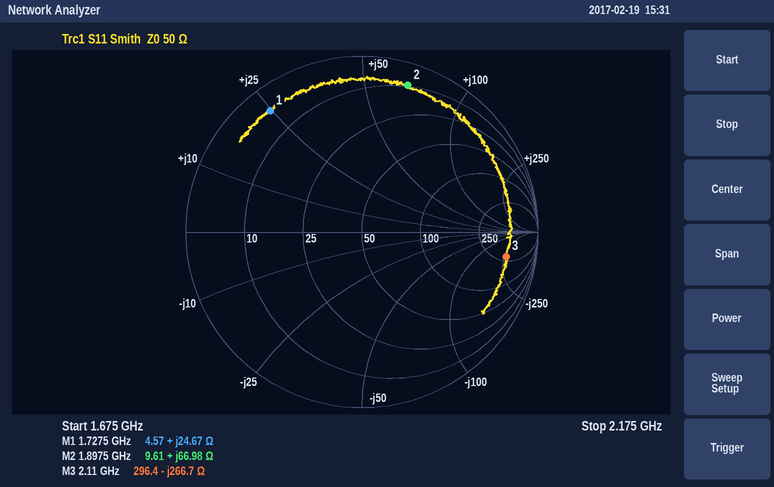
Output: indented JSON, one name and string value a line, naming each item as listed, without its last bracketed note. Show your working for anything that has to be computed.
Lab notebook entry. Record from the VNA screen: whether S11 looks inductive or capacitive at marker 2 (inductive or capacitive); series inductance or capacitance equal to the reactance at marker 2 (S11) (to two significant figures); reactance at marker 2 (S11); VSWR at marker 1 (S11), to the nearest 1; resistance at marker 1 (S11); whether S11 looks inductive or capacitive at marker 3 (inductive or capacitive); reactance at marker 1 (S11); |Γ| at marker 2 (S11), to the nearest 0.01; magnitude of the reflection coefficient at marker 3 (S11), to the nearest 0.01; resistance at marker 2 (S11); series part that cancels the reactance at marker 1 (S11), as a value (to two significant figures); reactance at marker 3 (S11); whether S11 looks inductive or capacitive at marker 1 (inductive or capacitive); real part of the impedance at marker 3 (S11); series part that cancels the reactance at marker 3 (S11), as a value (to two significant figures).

{
  "whether S11 looks inductive or capacitive at marker 2": "inductive",
  "series inductance or capacitance equal to the reactance at marker 2 (S11)": "L = 66.98 Ω/(2π × 1.8975 GHz) ≈ 5.6 nH",
  "reactance at marker 2": "+66.98 Ω",
  "VSWR at marker 1 (S11), to the nearest 1": "14",
  "resistance at marker 1": "4.57 Ω",
  "whether S11 looks inductive or capacitive at marker 3": "capacitive",
  "reactance at marker 1": "+24.67 Ω",
  "|Γ| at marker 2 (S11), to the nearest 0.01": "0.87",
  "magnitude of the reflection coefficient at marker 3 (S11), to the nearest 0.01": "0.83",
  "resistance at marker 2": "9.61 Ω",
  "series part that cancels the reactance at marker 1 (S11), as a value": "C = 1/(2π × 1.7275 GHz × 24.67 Ω) ≈ 3.7 pF",
  "reactance at marker 3": "-266.7 Ω",
  "whether S11 looks inductive or capacitive at marker 1": "inductive",
  "real part of the impedance at marker 3": "296.4 Ω",
  "series part that cancels the reactance at marker 3 (S11), as a value": "L = 266.7 Ω/(2π × 2.11 GHz) ≈ 20 nH"
}
